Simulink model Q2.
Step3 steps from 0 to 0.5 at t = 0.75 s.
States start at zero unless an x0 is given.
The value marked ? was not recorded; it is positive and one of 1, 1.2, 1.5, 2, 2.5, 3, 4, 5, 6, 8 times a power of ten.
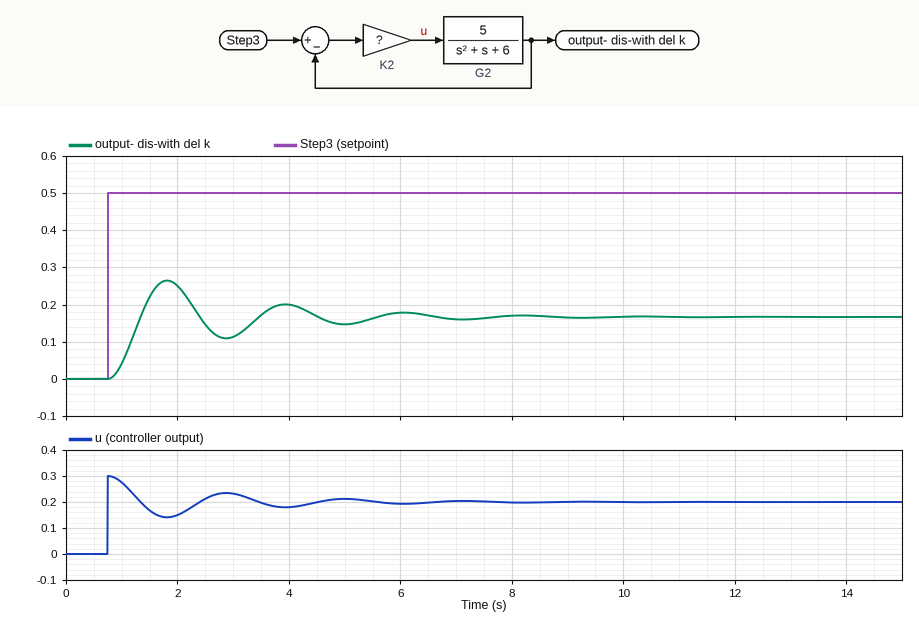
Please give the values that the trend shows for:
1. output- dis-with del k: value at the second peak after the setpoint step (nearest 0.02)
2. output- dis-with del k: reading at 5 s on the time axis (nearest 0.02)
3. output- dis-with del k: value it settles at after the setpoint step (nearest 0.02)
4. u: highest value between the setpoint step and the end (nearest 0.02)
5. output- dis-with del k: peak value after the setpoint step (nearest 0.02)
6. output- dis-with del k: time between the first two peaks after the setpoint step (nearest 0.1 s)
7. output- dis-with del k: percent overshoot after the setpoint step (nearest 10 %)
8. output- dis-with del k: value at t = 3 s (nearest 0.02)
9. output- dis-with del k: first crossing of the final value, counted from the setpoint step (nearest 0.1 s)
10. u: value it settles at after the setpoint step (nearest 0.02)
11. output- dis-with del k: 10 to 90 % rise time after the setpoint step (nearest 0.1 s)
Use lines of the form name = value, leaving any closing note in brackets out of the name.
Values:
output- dis-with del k: value at the second peak after the setpoint step = 0.20
output- dis-with del k: reading at 5 s on the time axis = 0.14
output- dis-with del k: value it settles at after the setpoint step = 0.16
u: highest value between the setpoint step and the end = 0.30
output- dis-with del k: peak value after the setpoint step = 0.26
output- dis-with del k: time between the first two peaks after the setpoint step = 2.1 s
output- dis-with del k: percent overshoot after the setpoint step = 60 %
output- dis-with del k: value at t = 3 s = 0.12
output- dis-with del k: first crossing of the final value, counted from the setpoint step = 0.6 s
u: value it settles at after the setpoint step = 0.20
output- dis-with del k: 10 to 90 % rise time after the setpoint step = 0.4 s
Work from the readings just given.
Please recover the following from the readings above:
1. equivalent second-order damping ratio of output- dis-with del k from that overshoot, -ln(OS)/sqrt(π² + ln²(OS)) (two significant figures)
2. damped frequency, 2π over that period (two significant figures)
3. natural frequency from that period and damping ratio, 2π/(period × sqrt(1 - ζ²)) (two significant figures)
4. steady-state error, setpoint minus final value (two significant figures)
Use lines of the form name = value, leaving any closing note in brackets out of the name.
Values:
equivalent second-order damping ratio of output- dis-with del k from that overshoot, -ln(OS)/sqrt(π² + ln²(OS)) = 0.16
damped frequency, 2π over that period = 3.0 rad/s
natural frequency from that period and damping ratio, 2π/(period × sqrt(1 - ζ²)) = 3.0 rad/s
steady-state error, setpoint minus final value = 0.34
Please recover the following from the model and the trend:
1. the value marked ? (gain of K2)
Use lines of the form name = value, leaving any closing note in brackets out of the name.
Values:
the value marked ? = 0.6
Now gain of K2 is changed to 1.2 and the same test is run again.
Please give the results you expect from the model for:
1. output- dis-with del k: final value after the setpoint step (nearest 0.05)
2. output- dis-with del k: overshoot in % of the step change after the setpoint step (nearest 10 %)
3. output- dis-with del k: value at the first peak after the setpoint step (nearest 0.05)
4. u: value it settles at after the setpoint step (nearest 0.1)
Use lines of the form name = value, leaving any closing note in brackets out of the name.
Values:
output- dis-with del k: final value after the setpoint step = 0.25
output- dis-with del k: overshoot in % of the step change after the setpoint step = 60 %
output- dis-with del k: value at the first peak after the setpoint step = 0.40
u: value it settles at after the setpoint step = 0.3
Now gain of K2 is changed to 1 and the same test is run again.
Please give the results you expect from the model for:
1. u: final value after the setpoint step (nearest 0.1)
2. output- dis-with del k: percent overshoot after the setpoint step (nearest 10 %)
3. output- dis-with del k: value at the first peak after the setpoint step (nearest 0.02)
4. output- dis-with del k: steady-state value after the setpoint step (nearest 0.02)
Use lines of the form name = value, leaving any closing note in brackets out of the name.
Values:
u: final value after the setpoint step = 0.3
output- dis-with del k: percent overshoot after the setpoint step = 60 %
output- dis-with del k: value at the first peak after the setpoint step = 0.36
output- dis-with del k: steady-state value after the setpoint step = 0.22
